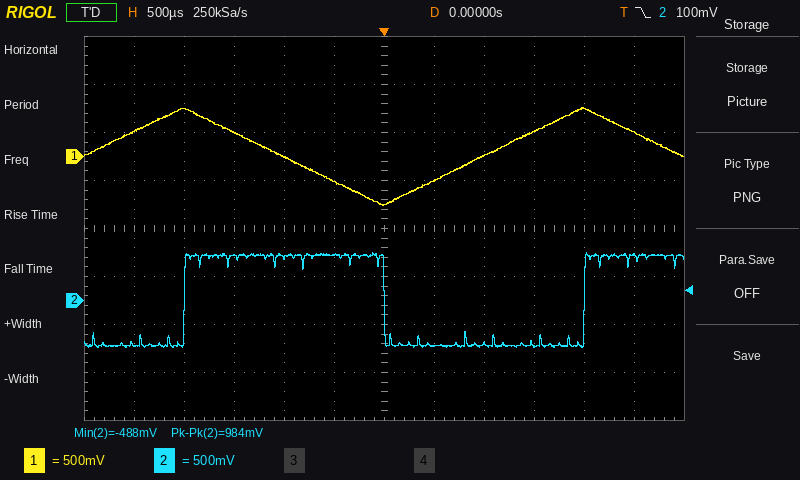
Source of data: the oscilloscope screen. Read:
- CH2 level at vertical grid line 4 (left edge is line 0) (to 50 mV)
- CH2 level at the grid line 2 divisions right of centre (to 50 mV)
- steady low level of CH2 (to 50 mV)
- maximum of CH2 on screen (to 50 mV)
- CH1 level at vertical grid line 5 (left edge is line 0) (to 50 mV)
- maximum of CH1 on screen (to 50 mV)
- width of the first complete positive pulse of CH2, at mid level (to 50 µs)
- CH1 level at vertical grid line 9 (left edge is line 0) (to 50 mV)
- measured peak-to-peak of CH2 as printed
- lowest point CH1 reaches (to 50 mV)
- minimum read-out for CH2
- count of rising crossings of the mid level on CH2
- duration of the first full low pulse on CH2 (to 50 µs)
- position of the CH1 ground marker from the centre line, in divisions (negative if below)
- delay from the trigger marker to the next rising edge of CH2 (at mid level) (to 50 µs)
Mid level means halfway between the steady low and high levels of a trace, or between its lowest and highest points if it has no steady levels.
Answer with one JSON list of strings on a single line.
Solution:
["450 mV", "-450 mV", "-450 mV", "500 mV", "-250 mV", "500 mV", "2.00 ms", "250 mV", "984 mV", "-500 mV", "-488 mV", "2", "2.00 ms", "+1.5 div", "2.00 ms"]
